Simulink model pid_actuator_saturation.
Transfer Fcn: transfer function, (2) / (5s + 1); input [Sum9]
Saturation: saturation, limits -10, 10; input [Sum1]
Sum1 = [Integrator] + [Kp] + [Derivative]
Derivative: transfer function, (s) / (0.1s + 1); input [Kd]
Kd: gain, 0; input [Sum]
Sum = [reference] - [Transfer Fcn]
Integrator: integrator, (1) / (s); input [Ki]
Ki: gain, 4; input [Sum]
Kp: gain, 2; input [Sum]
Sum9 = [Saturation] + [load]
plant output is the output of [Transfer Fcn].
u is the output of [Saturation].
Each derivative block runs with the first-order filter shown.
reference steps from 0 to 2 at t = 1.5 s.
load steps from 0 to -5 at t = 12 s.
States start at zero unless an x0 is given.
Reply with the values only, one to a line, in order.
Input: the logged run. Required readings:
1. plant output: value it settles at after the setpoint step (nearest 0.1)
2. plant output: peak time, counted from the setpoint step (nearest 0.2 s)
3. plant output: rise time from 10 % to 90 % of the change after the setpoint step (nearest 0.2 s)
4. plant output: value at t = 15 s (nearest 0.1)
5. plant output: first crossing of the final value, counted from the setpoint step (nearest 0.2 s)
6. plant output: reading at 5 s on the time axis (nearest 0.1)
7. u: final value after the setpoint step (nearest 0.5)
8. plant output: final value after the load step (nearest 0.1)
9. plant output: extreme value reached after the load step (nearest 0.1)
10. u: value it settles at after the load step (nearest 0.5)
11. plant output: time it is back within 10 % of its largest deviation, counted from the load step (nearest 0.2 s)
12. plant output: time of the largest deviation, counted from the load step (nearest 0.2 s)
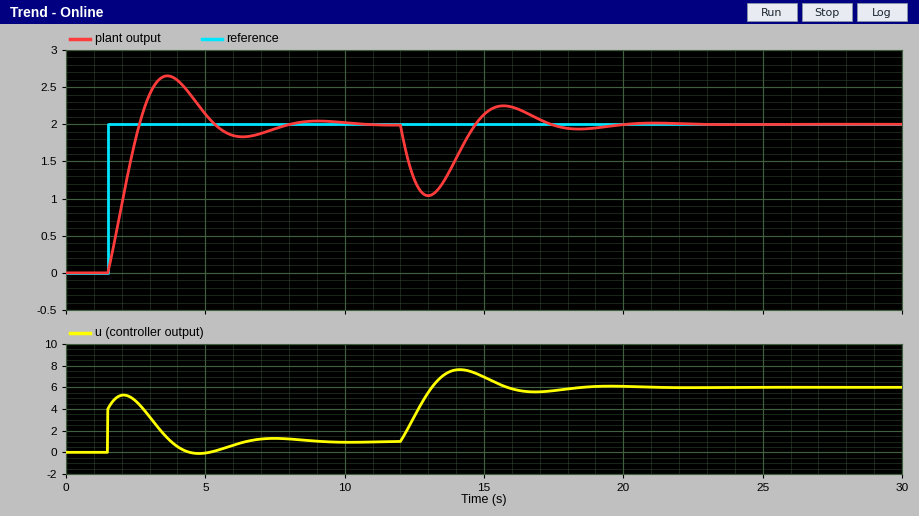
2.0
2.2 s
0.8 s
2.1
1.2 s
2.1
1.0
2.0
1.0
6.0
4.8 s
1.0 s
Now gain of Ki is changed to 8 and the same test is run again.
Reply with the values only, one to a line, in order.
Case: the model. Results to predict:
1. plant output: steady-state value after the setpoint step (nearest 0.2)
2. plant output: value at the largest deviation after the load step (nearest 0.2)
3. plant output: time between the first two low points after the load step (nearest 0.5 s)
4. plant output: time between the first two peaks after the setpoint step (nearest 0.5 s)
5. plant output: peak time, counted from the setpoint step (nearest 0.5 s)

2.0
1.2
3.5 s
3.5 s
1.5 s
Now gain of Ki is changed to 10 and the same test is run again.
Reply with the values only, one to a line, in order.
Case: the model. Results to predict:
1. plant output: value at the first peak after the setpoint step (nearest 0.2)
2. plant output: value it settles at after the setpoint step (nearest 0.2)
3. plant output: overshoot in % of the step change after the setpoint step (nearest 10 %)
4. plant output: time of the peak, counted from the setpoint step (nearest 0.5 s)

3.0
2.0
50 %
1.5 s
